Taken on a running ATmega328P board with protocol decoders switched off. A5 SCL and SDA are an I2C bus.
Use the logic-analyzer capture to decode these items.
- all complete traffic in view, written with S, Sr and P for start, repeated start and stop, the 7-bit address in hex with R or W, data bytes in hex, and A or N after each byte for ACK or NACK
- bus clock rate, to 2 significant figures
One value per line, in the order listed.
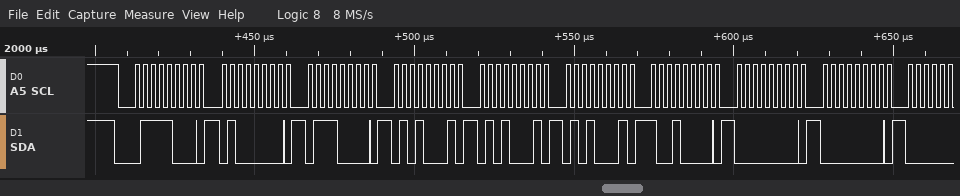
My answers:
S 3CW A 40 A 70 A 51 A 51 A 51 A 90 A 00 A 00 A
400 kHz
